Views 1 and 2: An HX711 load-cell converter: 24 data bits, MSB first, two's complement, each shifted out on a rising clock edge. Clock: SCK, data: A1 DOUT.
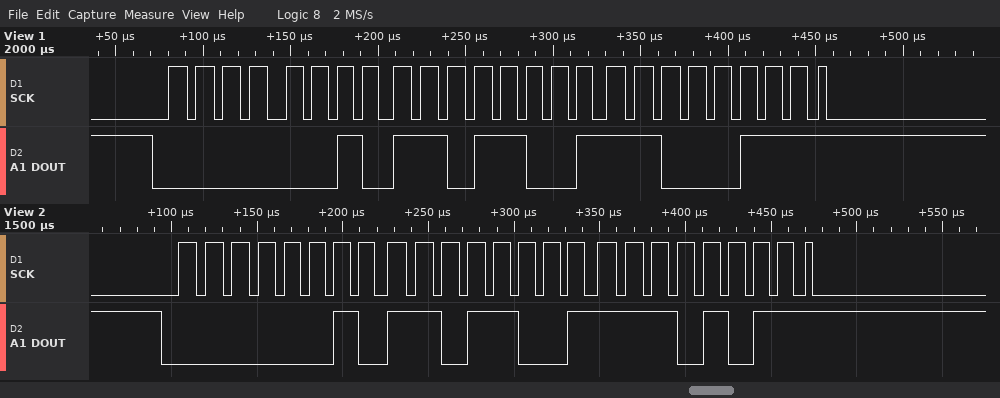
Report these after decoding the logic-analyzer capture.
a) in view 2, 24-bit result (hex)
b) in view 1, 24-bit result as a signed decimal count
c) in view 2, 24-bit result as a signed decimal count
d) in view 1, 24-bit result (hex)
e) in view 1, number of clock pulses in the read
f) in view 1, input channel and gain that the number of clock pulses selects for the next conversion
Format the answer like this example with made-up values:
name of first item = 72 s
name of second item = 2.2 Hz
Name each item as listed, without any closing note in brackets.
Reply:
in view 2, 24-bit result = 0x02D9EB
in view 1, 24-bit result as a signed decimal count = 186823
in view 2, 24-bit result as a signed decimal count = 186859
in view 1, 24-bit result = 0x02D9C7
in view 1, number of clock pulses in the read = 25
in view 1, input channel and gain that the number of clock pulses selects for the next conversion = channel A, gain 128
